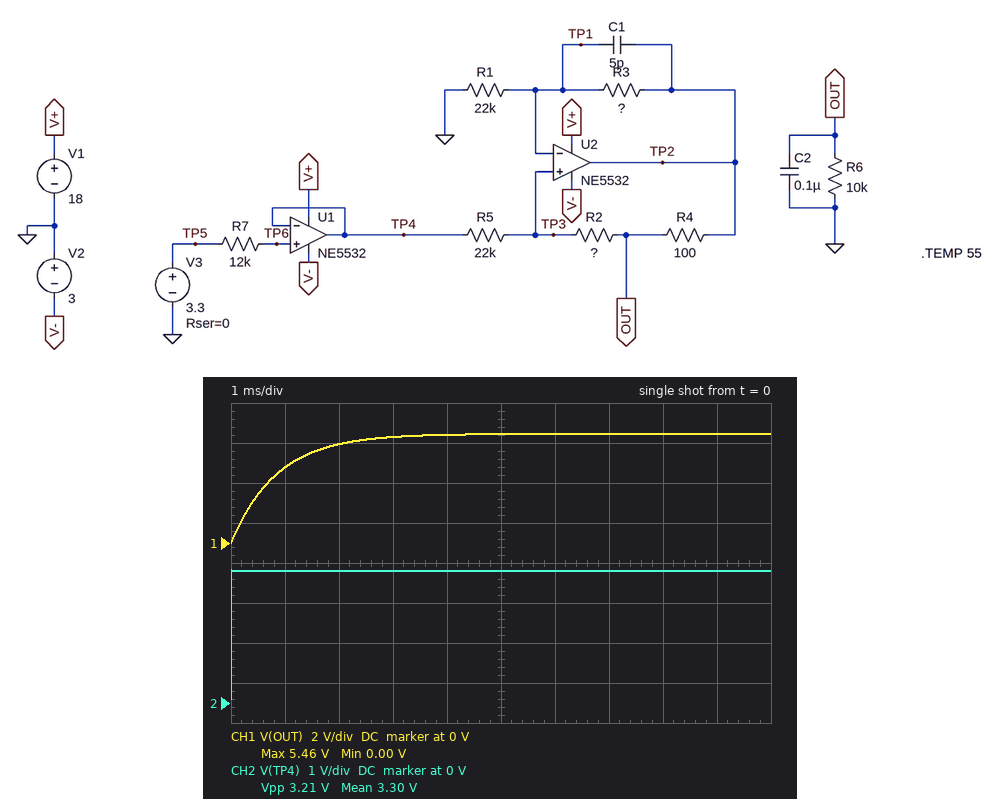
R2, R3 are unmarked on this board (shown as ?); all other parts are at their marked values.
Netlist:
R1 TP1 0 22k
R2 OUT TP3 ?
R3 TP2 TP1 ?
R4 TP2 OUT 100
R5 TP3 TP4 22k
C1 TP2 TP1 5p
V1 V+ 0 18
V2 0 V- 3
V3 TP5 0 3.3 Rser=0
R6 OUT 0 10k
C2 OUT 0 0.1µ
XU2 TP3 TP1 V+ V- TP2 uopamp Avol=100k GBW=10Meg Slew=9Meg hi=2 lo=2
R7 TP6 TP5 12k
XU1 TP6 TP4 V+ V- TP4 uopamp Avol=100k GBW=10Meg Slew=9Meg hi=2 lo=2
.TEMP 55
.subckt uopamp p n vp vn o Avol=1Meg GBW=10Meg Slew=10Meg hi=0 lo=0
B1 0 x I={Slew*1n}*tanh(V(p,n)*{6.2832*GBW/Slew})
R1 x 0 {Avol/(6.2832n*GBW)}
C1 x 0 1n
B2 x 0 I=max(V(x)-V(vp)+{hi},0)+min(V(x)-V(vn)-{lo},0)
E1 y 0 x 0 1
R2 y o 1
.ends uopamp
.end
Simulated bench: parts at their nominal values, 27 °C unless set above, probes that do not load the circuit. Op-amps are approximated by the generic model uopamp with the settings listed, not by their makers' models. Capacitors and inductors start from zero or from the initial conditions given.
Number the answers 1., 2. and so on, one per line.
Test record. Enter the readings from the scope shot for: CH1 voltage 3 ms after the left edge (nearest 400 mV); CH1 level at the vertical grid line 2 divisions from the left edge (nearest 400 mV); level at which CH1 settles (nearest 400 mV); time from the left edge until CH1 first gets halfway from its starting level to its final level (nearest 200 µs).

1. 5.2 V
2. 4.8 V
3. 5.6 V
4. 600 µs
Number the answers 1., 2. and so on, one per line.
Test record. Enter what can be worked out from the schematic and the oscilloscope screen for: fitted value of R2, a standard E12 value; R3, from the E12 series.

1. 330 Ω
2. 390 Ω
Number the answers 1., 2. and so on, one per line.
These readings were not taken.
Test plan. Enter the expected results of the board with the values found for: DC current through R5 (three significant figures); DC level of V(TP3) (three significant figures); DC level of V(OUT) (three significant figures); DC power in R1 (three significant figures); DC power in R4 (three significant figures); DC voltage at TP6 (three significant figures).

1. 96.6 µA
2. 5.43 V
3. 5.46 V
4. 1.34 mW
5. 41.3 µW
6. 3.30 V
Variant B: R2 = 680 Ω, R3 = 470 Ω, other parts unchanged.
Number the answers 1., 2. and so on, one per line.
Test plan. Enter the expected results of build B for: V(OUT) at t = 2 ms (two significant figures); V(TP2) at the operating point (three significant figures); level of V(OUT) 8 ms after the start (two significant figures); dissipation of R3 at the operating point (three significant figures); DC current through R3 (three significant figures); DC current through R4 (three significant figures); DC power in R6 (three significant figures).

1. 4.8 V
2. 4.94 V
3. 4.9 V
4. 22.7 µW
5. 220 µA
6. 558 µA
7. 2.38 mW
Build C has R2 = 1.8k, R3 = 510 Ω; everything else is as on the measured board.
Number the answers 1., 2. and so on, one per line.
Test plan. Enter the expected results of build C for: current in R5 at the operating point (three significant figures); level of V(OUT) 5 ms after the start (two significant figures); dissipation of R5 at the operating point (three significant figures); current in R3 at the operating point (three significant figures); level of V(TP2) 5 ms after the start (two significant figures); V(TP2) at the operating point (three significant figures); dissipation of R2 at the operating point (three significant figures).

1. 26.7 µA
2. 3.9 V
3. 15.7 µW
4. 177 µA
5. 4.0 V
6. 3.98 V
7. 1.28 µW
